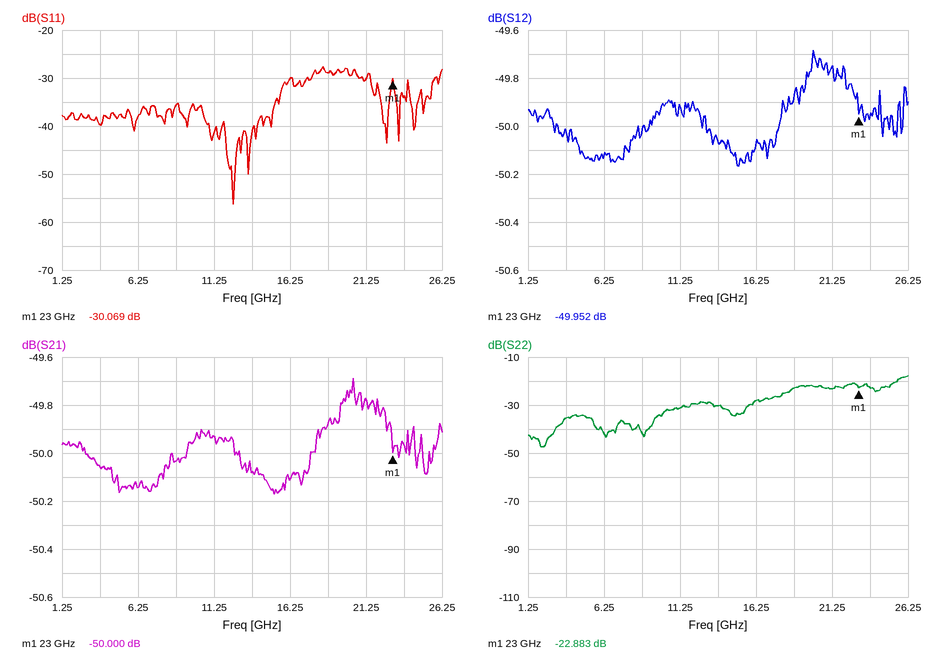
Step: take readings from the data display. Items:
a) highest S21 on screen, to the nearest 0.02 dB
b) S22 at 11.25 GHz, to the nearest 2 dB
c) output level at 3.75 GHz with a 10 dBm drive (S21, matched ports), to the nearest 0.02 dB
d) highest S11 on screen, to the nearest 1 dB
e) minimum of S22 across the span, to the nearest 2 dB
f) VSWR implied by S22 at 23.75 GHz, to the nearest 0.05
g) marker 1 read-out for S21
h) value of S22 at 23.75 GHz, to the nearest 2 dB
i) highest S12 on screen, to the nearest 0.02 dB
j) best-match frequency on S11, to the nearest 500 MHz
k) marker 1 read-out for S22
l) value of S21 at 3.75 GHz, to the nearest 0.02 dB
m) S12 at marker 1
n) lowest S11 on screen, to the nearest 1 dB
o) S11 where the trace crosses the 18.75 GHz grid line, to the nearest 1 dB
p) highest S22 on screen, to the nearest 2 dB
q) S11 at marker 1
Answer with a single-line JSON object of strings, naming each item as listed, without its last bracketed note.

{"highest S21 on screen, to the nearest 0.02 dB": "-49.68 dB", "S22 at 11.25 GHz, to the nearest 2 dB": "-32 dB", "output level at 3.75 GHz with a 10 dBm drive (S21, matched ports), to the nearest 0.02 dB": "-40.06 dBm", "highest S11 on screen, to the nearest 1 dB": "-28 dB", "minimum of S22 across the span, to the nearest 2 dB": "-48 dB", "VSWR implied by S22 at 23.75 GHz, to the nearest 0.05": "1.15", "marker 1 read-out for S21": "-50.000 dB", "value of S22 at 23.75 GHz, to the nearest 2 dB": "-22 dB", "highest S12 on screen, to the nearest 0.02 dB": "-49.68 dB", "best-match frequency on S11, to the nearest 500 MHz": "12.5 GHz", "marker 1 read-out for S22": "-22.883 dB", "value of S21 at 3.75 GHz, to the nearest 0.02 dB": "-50.06 dB", "S12 at marker 1": "-49.952 dB", "lowest S11 on screen, to the nearest 1 dB": "-56 dB", "S11 where the trace crosses the 18.75 GHz grid line, to the nearest 1 dB": "-29 dB", "highest S22 on screen, to the nearest 2 dB": "-18 dB", "S11 at marker 1": "-30.069 dB"}
